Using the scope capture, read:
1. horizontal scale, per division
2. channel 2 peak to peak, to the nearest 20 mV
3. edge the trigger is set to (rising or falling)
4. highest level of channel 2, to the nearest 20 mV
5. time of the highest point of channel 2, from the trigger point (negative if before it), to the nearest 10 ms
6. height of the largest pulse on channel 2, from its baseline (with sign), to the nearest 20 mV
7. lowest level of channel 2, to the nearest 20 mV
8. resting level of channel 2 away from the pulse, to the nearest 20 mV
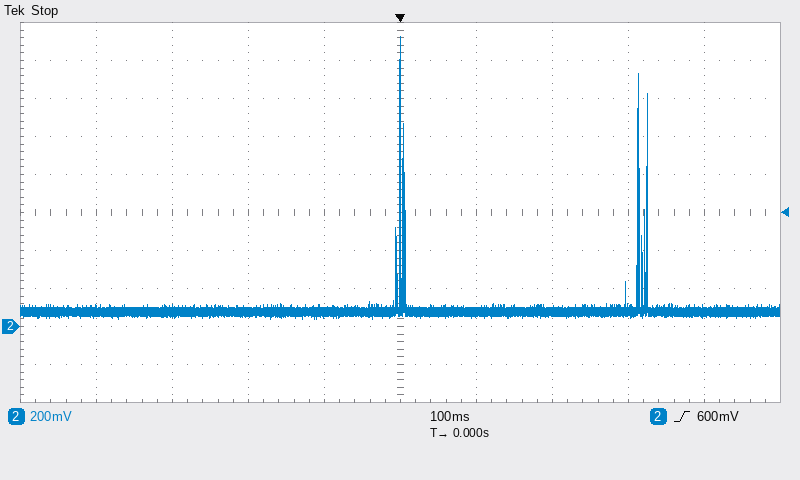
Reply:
100 ms
1.48 V
rising
1.52 V
0 ms
+1.44 V
40 mV
80 mV
